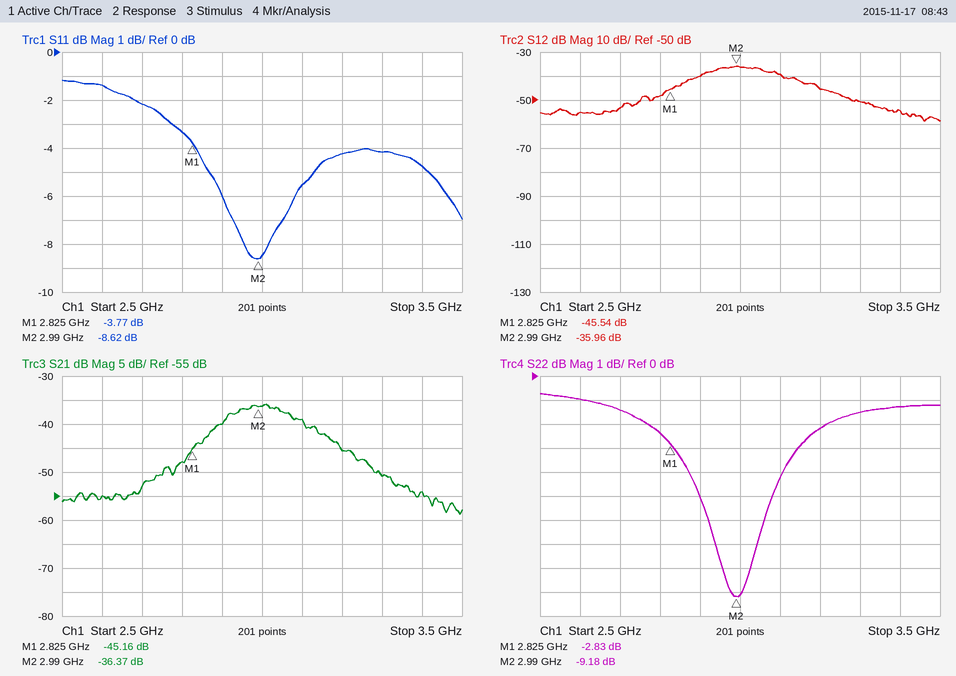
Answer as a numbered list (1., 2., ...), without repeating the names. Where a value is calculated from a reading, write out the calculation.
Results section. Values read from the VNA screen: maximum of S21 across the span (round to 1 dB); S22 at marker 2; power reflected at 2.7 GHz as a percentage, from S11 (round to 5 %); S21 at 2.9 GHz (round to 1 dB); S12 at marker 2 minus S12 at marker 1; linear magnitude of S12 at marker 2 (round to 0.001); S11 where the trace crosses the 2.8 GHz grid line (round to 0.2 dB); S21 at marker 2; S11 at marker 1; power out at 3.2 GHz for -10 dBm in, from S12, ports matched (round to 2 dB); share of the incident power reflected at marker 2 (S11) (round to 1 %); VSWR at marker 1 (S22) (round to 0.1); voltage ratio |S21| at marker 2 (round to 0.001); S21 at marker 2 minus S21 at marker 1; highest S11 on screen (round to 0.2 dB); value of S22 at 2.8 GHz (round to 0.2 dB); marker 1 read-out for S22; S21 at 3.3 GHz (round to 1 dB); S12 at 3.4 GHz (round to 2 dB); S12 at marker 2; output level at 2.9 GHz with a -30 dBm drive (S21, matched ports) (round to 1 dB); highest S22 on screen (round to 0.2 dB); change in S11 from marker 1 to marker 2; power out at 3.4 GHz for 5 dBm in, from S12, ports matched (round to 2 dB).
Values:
1. -36 dB
2. -9.18 dB
3. 10^(-2.2/10) ≈ 60 %
4. -40 dB
5. -35.96 − (-45.54) = 9.58 dB
6. 10^(-35.96/20) ≈ 0.016
7. -3.4 dB
8. -36.37 dB
9. -3.77 dB
10. -10 dBm + (-46 dB) = -56 dBm
11. 10^(-8.62/10) ≈ 14 %
12. (1 + 0.7219)/(1 − 0.7219) ≈ 6.2
13. 10^(-36.37/20) ≈ 0.015
14. -36.37 − (-45.16) = 8.79 dB
15. -1.2 dB
16. -2.4 dB
17. -2.83 dB
18. -51 dB
19. -54 dB
20. -35.96 dB
21. -30 dBm + (-40 dB) = -70 dBm
22. -0.8 dB
23. -8.62 − (-3.77) = -4.85 dB
24. 5 dBm + (-54 dB) = -50 dBm
